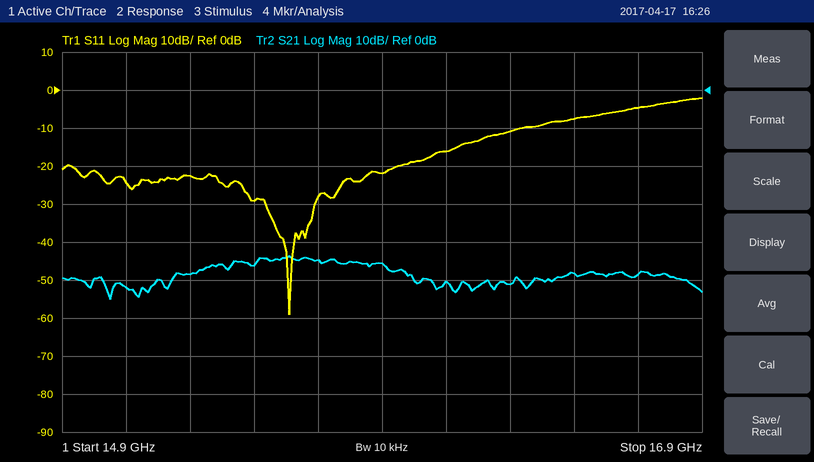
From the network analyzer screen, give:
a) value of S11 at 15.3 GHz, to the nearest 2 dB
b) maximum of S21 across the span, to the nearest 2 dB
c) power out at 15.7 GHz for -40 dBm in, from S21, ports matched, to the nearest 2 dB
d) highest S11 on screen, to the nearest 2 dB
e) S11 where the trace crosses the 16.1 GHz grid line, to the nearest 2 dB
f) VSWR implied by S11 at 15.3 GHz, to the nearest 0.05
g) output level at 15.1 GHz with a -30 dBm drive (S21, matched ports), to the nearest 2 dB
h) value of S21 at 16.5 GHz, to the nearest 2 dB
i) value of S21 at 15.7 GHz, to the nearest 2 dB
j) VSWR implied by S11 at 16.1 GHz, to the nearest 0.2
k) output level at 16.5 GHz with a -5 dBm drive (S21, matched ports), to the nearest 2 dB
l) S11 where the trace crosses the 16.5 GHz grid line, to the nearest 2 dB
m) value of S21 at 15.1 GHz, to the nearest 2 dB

-22 dB
-44 dB
-84 dBm
-2 dB
-16 dB
1.15
-82 dBm
-48 dB
-44 dB
1.4
-54 dBm
-8 dB
-52 dB
